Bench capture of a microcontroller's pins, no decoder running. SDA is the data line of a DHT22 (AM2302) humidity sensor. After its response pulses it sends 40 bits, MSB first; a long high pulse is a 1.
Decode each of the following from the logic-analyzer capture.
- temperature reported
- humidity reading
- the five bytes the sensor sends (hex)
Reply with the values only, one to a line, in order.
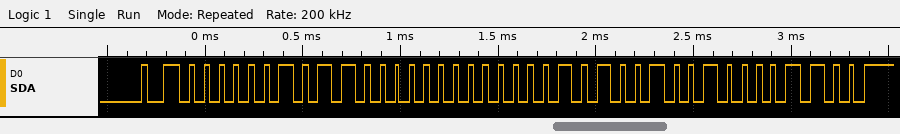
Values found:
32.9 °C
70.4 %
02 C0 01 49 0C
